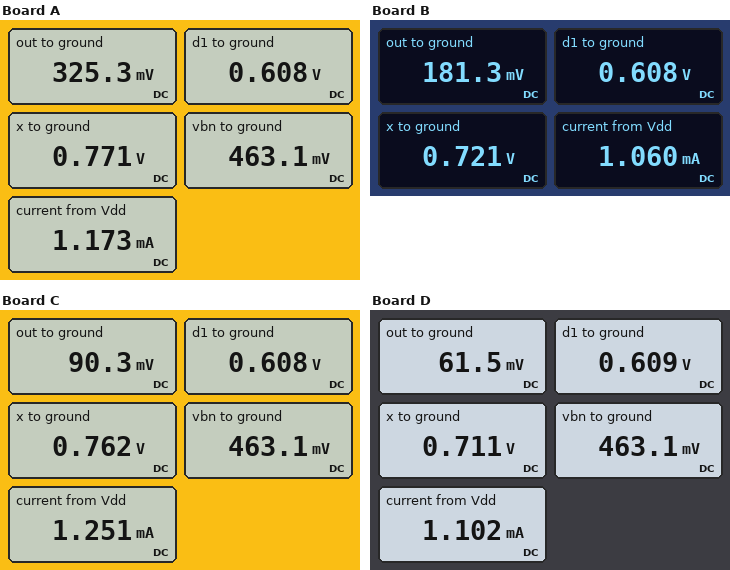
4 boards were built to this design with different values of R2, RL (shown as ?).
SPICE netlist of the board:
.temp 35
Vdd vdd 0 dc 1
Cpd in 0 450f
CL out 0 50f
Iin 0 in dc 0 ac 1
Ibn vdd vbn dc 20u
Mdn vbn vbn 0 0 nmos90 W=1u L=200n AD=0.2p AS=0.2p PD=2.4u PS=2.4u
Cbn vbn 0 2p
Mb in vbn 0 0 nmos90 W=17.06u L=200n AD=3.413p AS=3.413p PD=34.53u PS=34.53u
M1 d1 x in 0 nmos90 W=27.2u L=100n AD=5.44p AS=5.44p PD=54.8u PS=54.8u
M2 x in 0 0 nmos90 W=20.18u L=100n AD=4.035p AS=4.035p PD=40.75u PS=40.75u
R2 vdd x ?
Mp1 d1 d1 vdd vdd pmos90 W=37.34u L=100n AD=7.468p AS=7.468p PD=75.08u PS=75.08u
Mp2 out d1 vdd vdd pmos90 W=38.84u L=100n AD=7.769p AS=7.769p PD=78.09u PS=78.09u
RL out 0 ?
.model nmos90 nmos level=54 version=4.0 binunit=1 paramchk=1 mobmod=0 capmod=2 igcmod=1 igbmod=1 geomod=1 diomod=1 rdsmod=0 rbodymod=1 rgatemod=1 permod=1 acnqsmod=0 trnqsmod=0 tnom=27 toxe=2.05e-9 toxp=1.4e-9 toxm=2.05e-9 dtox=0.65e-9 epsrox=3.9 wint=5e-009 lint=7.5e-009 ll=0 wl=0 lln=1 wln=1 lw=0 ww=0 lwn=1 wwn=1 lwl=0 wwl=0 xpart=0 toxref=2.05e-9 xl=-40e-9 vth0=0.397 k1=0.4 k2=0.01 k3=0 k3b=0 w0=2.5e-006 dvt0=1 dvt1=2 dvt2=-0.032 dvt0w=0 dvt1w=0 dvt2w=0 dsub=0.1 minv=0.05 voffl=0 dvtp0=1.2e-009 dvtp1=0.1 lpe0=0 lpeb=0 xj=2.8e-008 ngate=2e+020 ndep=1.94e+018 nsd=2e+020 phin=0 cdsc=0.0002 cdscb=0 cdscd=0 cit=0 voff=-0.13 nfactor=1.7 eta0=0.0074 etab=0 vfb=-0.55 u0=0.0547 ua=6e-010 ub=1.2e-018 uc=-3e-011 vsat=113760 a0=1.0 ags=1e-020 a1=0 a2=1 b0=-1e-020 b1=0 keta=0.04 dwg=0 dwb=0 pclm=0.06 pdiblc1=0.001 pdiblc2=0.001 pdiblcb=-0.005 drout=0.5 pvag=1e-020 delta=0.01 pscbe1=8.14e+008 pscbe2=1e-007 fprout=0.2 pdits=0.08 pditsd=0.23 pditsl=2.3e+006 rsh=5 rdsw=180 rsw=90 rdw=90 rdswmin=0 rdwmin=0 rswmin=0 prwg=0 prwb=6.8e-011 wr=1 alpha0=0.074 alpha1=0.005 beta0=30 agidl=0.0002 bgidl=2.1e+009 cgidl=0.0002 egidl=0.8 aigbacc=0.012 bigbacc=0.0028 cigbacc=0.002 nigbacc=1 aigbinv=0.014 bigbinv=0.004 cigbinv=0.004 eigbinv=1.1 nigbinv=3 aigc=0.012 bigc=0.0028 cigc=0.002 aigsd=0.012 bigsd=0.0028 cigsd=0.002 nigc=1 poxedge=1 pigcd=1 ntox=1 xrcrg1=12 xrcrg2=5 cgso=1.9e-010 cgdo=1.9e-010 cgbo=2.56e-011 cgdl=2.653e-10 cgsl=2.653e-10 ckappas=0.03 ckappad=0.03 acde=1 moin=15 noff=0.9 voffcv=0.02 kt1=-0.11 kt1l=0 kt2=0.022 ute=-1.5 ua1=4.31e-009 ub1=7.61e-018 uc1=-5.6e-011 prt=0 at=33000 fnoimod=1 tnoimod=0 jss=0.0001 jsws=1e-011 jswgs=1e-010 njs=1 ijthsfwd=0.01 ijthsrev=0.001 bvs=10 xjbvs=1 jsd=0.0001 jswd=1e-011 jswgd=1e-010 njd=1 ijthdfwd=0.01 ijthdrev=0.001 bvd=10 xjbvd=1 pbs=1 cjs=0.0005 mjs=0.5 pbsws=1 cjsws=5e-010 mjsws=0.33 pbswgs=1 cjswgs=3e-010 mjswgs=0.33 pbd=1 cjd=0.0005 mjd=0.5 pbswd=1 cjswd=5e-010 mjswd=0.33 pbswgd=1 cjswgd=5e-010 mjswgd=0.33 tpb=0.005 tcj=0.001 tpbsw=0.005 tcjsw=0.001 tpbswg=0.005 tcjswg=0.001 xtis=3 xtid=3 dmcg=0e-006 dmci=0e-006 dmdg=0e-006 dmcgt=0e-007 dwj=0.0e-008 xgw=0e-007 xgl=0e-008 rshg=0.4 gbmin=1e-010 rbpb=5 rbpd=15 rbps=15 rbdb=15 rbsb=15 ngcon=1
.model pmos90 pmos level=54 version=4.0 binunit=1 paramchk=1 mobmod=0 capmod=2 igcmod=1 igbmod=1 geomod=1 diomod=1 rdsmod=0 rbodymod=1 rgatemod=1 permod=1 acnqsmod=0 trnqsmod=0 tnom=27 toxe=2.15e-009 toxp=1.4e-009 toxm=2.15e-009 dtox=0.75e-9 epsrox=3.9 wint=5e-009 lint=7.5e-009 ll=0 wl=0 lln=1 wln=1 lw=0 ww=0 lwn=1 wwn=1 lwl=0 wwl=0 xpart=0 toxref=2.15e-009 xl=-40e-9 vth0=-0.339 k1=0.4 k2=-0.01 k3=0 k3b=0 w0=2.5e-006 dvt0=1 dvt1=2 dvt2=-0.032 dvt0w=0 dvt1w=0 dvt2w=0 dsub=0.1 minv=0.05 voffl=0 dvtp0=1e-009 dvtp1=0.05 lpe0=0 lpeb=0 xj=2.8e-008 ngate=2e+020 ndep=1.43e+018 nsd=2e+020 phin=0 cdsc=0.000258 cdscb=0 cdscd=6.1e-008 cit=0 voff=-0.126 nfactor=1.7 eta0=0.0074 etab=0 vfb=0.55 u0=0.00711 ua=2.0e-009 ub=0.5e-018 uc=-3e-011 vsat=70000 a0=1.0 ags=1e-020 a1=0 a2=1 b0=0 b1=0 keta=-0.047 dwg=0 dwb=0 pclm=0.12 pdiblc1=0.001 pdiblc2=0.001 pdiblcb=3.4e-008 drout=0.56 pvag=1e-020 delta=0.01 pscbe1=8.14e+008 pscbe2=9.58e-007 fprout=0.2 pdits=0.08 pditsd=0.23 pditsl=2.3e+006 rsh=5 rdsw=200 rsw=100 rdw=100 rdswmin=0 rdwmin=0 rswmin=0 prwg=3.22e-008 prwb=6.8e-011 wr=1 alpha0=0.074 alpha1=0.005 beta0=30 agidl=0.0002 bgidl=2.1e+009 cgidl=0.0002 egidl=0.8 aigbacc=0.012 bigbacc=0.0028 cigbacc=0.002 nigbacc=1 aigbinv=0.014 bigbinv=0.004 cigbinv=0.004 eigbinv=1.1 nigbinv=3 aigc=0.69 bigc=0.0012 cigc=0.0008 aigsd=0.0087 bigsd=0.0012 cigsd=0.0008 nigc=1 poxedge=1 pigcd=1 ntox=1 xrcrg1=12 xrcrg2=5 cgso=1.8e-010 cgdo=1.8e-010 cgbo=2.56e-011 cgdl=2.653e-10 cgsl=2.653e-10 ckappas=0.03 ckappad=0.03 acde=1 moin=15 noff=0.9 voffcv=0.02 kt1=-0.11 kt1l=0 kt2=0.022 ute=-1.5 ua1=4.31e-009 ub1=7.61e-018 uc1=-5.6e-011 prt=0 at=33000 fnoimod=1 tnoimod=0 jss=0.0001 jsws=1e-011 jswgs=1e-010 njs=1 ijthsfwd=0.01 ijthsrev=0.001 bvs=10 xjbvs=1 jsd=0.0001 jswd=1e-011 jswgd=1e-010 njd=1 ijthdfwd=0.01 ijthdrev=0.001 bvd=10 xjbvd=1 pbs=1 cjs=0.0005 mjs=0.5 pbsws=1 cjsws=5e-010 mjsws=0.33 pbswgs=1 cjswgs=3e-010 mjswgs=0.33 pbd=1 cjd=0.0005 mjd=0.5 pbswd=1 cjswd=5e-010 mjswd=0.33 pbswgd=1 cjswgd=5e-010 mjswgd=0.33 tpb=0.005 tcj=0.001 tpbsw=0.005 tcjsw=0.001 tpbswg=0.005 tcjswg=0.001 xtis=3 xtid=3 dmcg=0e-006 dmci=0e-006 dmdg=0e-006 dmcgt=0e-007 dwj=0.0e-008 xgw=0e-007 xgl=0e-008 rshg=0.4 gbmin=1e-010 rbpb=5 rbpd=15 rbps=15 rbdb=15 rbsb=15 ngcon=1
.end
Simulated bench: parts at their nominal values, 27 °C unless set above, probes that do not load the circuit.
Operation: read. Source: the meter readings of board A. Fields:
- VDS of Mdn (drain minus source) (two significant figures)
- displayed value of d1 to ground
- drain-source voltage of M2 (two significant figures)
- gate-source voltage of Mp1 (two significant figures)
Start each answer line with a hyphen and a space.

- 460 mV
- 0.608 V
- 770 mV
- -390 mV
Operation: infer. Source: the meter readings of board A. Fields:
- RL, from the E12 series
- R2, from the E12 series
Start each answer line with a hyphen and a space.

- 680 Ω
- 680 Ω
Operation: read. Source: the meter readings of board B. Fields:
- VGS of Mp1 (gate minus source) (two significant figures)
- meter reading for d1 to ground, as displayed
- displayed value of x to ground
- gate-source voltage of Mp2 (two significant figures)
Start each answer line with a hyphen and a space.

- -390 mV
- 0.608 V
- 0.721 V
- -390 mV
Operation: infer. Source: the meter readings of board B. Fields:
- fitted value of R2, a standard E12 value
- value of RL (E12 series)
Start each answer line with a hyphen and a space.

- 1.8 kΩ
- 330 Ω
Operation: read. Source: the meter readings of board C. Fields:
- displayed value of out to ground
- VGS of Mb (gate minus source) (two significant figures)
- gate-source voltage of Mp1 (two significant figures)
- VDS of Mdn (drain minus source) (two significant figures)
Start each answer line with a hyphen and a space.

- 90.3 mV
- 460 mV
- -390 mV
- 460 mV
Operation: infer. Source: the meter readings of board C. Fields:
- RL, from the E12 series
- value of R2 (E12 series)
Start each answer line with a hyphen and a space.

- 150 Ω
- 820 Ω
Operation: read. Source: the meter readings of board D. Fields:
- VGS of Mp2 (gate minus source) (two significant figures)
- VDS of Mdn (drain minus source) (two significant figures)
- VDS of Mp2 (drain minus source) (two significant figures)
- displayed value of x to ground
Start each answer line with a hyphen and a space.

- -390 mV
- 460 mV
- -940 mV
- 0.711 V
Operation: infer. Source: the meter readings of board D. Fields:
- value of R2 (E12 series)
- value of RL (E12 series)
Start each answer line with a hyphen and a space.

- 2.2 kΩ
- 100 Ω
